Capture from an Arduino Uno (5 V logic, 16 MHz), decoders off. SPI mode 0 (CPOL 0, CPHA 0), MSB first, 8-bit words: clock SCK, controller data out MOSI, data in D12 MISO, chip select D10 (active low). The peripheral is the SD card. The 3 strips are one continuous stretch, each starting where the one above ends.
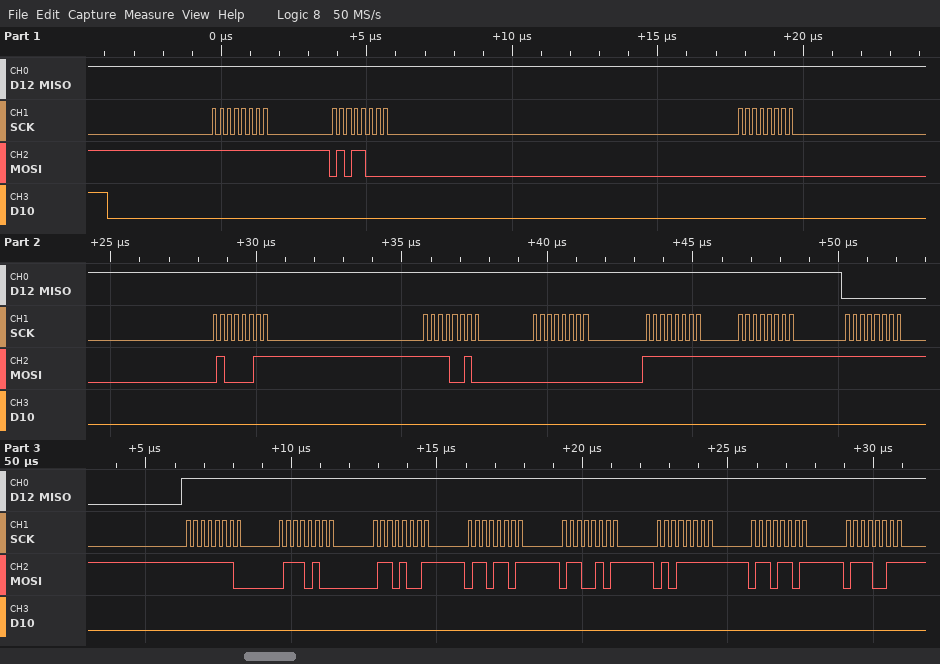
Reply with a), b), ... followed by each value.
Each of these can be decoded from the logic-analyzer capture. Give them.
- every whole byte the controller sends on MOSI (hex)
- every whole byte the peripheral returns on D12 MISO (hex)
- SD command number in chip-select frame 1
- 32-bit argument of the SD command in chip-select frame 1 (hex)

a) FF 58 00 43 F2 00 FF FF FF FE 74 69 6D 65 5F 6D 73
b) FF FF FF FF FF FF FF FF 00 FF FF FF FF FF FF FF FF
c) CMD24
d) 0x0043F200
